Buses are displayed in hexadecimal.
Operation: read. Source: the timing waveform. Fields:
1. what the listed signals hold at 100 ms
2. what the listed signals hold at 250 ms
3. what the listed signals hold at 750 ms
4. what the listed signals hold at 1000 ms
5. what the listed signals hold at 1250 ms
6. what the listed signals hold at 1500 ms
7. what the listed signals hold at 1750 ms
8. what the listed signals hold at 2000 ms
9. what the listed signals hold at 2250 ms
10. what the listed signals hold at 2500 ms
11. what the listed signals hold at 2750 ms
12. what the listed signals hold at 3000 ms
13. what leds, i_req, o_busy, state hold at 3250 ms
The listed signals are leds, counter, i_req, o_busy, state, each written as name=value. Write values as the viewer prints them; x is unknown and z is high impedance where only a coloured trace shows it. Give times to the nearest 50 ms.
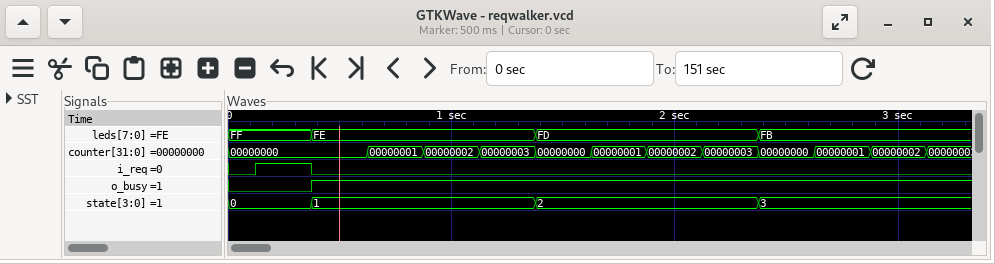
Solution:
leds=FF, counter=00000000, i_req=0, o_busy=0, state=0
leds=FF, counter=00000000, i_req=1, o_busy=0, state=0
leds=FE, counter=00000001, i_req=0, o_busy=1, state=1
leds=FE, counter=00000002, i_req=0, o_busy=1, state=1
leds=FE, counter=00000003, i_req=0, o_busy=1, state=1
leds=FD, counter=00000000, i_req=0, o_busy=1, state=2
leds=FD, counter=00000001, i_req=0, o_busy=1, state=2
leds=FD, counter=00000002, i_req=0, o_busy=1, state=2
leds=FD, counter=00000003, i_req=0, o_busy=1, state=2
leds=FB, counter=00000000, i_req=0, o_busy=1, state=3
leds=FB, counter=00000001, i_req=0, o_busy=1, state=3
leds=FB, counter=00000002, i_req=0, o_busy=1, state=3
leds=FB, i_req=0, o_busy=1, state=3
